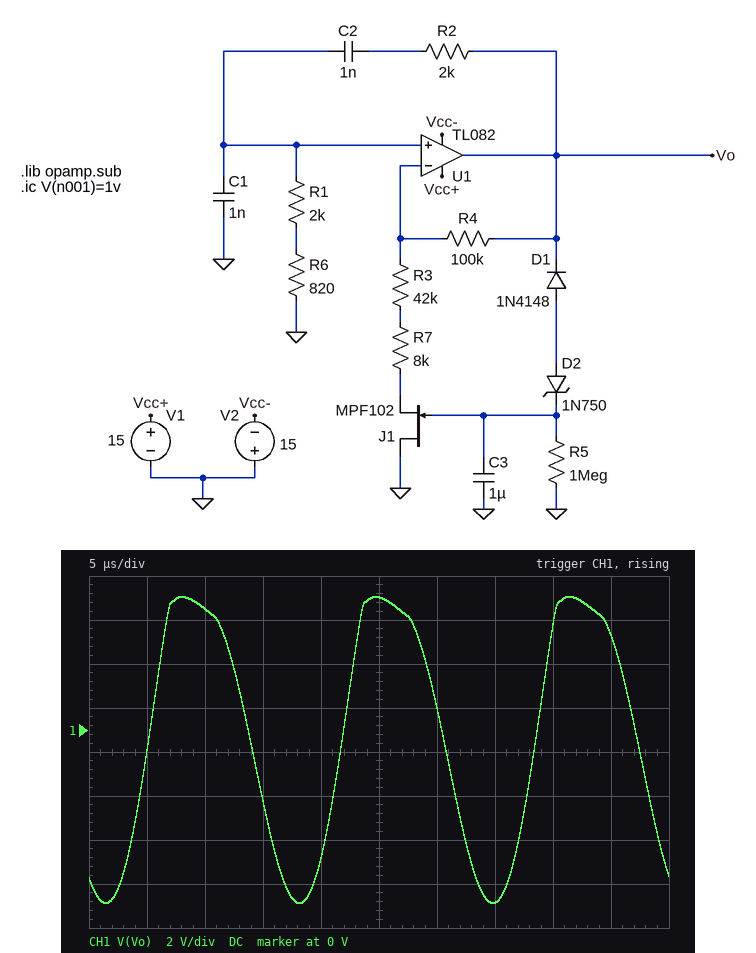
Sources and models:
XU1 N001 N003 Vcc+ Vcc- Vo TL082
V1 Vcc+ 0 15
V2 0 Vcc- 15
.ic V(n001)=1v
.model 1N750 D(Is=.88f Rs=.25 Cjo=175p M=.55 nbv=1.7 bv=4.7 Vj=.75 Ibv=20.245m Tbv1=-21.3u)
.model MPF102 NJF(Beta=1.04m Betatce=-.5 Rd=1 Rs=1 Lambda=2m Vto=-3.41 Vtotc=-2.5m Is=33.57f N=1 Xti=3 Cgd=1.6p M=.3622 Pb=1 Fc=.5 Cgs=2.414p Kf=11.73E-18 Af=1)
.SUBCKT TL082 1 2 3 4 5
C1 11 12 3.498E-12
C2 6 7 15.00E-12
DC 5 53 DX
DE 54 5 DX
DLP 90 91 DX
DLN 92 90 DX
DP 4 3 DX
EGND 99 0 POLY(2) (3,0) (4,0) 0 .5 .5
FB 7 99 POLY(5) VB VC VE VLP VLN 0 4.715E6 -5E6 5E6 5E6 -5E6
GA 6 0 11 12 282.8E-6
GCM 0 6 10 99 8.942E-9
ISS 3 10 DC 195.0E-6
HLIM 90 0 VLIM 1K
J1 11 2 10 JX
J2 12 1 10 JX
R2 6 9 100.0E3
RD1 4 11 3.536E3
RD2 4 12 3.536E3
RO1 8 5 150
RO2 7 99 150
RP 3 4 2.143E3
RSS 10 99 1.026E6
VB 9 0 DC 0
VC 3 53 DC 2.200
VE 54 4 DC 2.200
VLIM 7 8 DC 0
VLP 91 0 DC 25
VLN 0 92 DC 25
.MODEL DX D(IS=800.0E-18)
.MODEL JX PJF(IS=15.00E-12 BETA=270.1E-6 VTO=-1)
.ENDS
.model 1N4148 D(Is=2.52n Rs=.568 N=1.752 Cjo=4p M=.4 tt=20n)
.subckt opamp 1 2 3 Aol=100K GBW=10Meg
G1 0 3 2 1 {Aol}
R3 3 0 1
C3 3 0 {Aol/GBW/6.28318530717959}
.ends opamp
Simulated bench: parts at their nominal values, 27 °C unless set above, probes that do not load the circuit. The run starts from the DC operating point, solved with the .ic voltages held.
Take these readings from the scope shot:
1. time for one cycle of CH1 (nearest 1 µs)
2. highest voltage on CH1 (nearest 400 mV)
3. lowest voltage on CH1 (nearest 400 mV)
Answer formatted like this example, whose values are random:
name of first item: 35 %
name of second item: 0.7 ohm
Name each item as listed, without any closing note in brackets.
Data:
time for one cycle of CH1: 17 µs
highest voltage on CH1: 6.0 V
lowest voltage on CH1: -8.0 V
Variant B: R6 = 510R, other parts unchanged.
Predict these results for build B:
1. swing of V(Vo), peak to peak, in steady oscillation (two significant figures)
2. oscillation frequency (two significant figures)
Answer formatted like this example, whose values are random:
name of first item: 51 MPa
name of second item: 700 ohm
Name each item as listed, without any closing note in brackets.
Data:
swing of V(Vo), peak to peak, in steady oscillation: 15 V
oscillation frequency: 64 kHz
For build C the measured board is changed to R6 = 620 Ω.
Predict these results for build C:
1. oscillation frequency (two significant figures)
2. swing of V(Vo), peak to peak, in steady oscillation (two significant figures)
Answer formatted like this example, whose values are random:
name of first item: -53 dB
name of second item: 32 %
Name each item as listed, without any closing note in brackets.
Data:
oscillation frequency: 63 kHz
swing of V(Vo), peak to peak, in steady oscillation: 12 V
